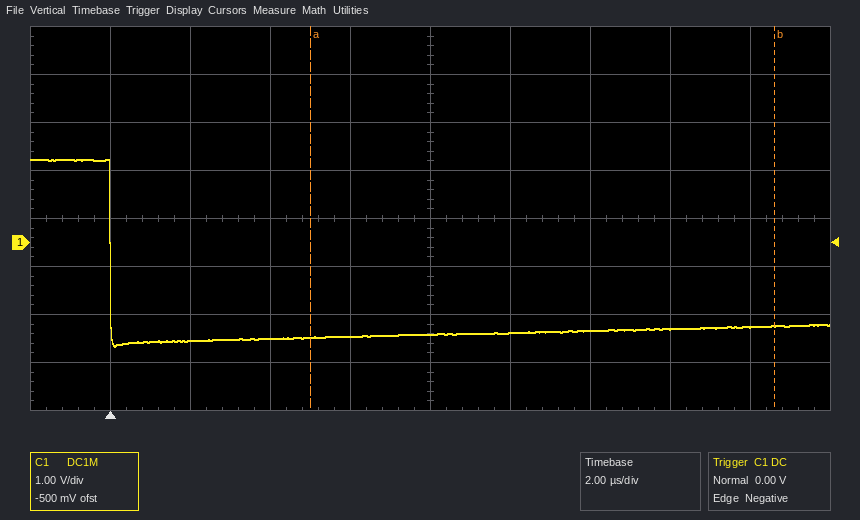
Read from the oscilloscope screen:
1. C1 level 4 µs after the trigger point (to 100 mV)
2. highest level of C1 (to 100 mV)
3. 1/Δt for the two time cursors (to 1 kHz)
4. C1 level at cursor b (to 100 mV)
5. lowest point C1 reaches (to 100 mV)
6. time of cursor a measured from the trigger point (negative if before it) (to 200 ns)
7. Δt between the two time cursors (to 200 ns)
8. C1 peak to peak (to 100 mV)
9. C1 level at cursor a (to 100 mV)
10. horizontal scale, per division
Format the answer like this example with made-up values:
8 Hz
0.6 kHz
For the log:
-2.0 V
1.7 V
86 kHz
-1.7 V
-2.2 V
+5.0 µs
11.6 µs
3.9 V
-2.0 V
2 µs
